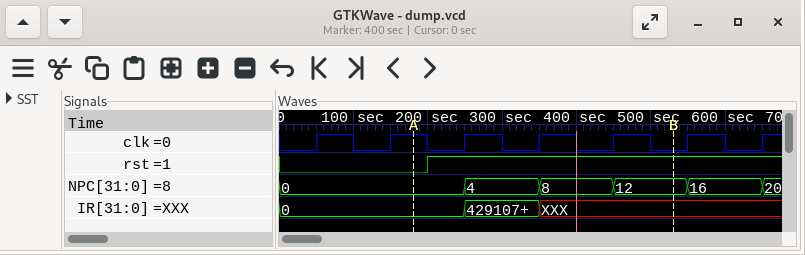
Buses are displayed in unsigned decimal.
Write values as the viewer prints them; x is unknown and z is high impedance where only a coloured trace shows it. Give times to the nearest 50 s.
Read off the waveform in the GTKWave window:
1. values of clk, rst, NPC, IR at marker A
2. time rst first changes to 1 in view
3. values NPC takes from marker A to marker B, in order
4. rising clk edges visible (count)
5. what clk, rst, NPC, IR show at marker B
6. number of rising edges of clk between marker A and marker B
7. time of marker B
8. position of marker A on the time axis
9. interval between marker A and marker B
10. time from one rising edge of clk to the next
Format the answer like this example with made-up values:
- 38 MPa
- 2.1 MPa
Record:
- clk=1, rst=0, NPC=0, IR=0
- 200 s
- 0, 4, 8, 12
- 7
- clk=0, rst=1, NPC=12, IR=XXX
- 3
- 550 s
- 200 s
- 350 s
- 100 s
